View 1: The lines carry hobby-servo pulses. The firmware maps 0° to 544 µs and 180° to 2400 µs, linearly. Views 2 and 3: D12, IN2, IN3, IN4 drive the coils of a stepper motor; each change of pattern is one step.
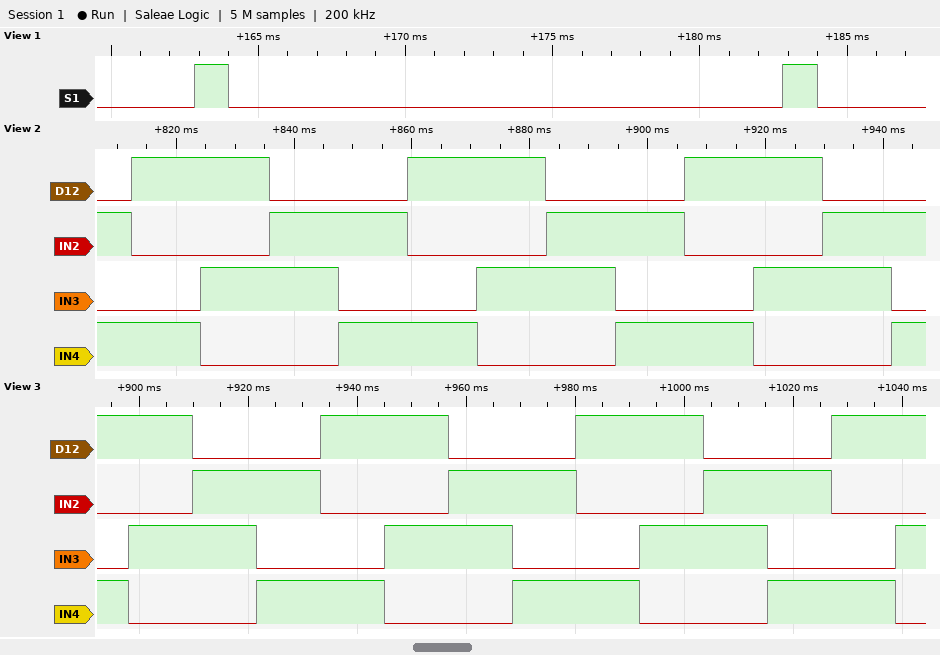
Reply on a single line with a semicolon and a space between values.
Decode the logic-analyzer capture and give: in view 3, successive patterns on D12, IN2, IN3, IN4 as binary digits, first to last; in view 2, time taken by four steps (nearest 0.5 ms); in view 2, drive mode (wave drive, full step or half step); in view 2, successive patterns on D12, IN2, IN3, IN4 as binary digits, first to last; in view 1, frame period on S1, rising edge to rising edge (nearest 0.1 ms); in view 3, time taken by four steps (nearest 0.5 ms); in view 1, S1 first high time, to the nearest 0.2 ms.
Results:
1001 1010 0110 0101 1001 1010 0110 0101 1001 1010 0110 0101 1001 1010; 47.0 ms; full step; 0101 1001 1010 0110 0101 1001 1010 0110 0101 1001 1010 0110 0101; 20.0 ms; 47.0 ms; 1.2 ms
